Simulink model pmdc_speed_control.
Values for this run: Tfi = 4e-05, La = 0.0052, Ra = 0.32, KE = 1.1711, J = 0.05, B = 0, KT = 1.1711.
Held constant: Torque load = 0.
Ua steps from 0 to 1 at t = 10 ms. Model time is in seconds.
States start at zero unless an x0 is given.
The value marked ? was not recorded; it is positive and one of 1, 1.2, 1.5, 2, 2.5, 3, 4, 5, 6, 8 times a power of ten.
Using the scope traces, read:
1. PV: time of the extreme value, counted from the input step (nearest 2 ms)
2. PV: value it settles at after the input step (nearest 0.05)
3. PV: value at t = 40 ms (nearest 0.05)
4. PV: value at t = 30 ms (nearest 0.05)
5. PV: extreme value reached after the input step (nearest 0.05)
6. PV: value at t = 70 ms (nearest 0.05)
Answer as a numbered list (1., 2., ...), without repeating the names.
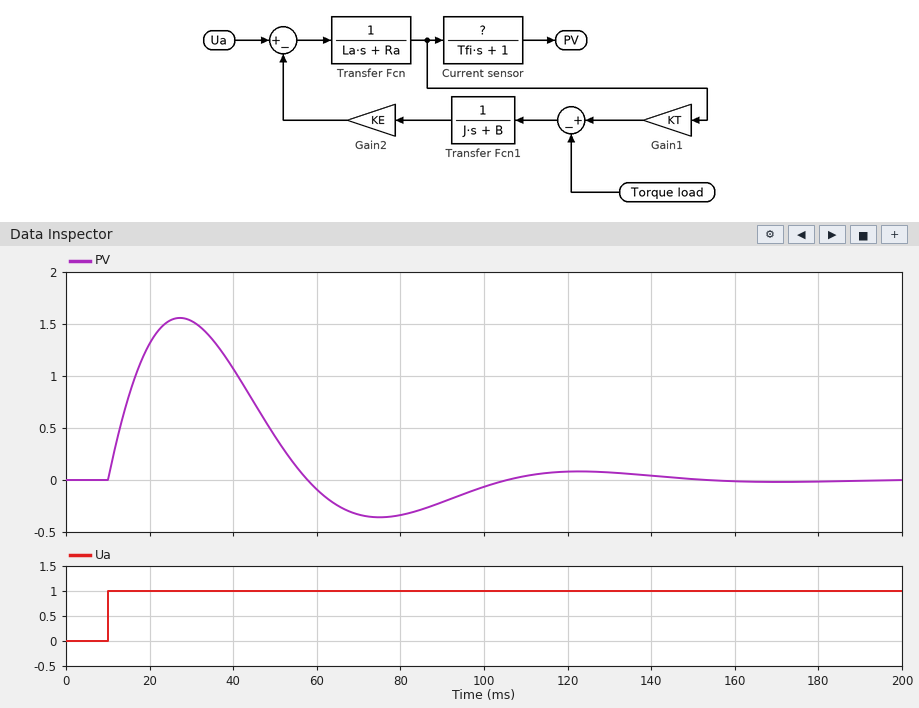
1. 18 ms
2. 0.00
3. 1.05
4. 1.55
5. 1.55
6. -0.35
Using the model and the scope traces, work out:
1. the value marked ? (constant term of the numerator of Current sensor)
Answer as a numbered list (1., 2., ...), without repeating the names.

1. 1
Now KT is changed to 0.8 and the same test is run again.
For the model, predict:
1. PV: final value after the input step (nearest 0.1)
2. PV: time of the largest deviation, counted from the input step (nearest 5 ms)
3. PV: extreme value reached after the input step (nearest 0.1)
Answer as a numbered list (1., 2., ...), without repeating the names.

1. 0.0
2. 20 ms
3. 1.7
